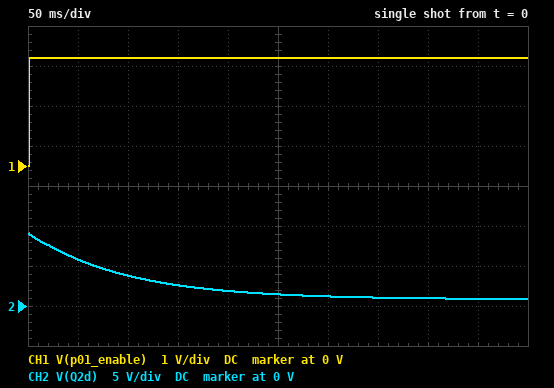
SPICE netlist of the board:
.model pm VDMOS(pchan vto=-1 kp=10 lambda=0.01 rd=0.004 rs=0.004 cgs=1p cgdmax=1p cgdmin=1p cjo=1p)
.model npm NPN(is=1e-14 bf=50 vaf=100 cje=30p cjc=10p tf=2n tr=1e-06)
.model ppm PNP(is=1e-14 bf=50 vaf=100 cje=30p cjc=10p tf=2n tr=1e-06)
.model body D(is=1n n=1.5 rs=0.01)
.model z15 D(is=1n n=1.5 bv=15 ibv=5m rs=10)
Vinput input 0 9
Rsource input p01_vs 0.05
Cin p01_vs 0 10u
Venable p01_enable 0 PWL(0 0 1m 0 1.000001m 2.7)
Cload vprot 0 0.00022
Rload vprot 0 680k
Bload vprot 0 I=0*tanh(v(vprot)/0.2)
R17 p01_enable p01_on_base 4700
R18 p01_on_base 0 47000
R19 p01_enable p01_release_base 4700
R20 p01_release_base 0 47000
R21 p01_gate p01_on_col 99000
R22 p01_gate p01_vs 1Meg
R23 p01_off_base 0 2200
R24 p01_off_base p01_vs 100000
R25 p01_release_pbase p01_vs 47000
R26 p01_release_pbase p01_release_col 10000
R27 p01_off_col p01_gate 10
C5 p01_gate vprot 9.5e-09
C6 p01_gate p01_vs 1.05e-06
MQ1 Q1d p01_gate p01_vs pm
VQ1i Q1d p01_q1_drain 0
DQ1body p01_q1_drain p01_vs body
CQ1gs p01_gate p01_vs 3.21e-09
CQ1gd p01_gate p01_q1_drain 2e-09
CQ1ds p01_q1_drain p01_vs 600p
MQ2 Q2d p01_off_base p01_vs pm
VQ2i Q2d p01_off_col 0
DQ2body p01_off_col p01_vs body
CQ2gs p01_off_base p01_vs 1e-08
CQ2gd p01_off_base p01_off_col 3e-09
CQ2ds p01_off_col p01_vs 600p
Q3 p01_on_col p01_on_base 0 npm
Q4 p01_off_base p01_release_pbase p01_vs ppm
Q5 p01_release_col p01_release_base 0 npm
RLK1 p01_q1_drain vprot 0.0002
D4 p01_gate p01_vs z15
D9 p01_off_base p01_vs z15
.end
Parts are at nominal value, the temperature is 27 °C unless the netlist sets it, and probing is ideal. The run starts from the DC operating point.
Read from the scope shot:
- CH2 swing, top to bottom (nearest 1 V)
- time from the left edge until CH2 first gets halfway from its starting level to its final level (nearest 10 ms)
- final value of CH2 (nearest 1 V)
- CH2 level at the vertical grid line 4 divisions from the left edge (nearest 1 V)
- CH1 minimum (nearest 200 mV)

8 V
70 ms
1 V
2 V
0 V
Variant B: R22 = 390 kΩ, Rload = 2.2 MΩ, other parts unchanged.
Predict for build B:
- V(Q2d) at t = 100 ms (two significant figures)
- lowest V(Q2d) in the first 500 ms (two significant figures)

4.1 V
1.9 V
